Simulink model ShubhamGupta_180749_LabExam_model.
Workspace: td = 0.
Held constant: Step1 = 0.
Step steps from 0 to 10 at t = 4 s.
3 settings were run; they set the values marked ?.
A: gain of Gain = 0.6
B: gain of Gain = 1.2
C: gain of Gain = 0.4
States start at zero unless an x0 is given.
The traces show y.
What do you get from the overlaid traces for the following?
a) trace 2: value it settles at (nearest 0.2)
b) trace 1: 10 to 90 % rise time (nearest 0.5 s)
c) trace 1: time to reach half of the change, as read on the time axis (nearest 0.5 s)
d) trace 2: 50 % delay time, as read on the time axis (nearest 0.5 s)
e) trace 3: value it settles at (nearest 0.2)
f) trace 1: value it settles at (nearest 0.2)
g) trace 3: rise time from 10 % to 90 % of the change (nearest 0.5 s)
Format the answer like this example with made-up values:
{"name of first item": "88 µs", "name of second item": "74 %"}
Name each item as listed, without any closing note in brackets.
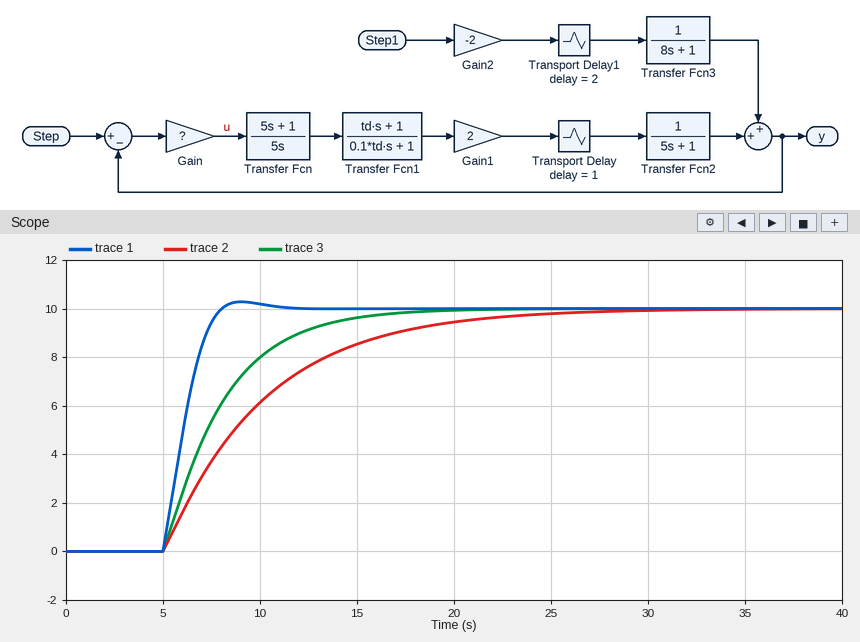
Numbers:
{"trace 2: value it settles at": "10.0", "trace 1: 10 to 90 % rise time": "2.0 s", "trace 1: time to reach half of the change, as read on the time axis": "6.0 s", "trace 2: 50 % delay time, as read on the time axis": "8.5 s", "trace 3: value it settles at": "10.0", "trace 1: value it settles at": "10.0", "trace 3: rise time from 10 % to 90 % of the change": "6.5 s"}
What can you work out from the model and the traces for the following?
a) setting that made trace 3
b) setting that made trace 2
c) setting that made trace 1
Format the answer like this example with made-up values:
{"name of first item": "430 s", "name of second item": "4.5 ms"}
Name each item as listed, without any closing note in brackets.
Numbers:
{"setting that made trace 3": "A", "setting that made trace 2": "C", "setting that made trace 1": "B"}
